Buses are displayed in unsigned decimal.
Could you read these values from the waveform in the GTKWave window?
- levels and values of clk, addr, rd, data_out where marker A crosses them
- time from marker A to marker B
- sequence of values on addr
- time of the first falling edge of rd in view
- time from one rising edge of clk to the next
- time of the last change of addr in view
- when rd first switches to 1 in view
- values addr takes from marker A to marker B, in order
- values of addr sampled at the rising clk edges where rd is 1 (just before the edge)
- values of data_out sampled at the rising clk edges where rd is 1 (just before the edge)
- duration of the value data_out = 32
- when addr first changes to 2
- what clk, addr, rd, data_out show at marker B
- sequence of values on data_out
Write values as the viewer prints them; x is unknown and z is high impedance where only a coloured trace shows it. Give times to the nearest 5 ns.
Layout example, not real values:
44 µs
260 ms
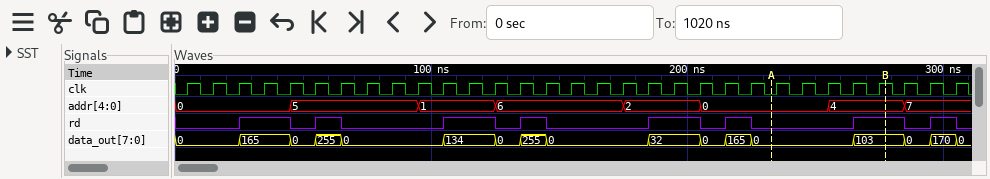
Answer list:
clk=0, addr=0, rd=0, data_out=0
45 ns
0, 5, 1, 6, 2, 0, 4, 7
45 ns
10 ns
285 ns
25 ns
0, 4
0, 0, 5, 1, 1, 6, 2, 2, 0, 4, 4, 7
165, 165, 255, 134, 134, 255, 32, 32, 165, 103, 103, 170
20 ns
175 ns
clk=1, addr=4, rd=1, data_out=103
0, 165, 0, 255, 0, 134, 0, 255, 0, 32, 0, 165, 0, 103, 0, 170, 0
